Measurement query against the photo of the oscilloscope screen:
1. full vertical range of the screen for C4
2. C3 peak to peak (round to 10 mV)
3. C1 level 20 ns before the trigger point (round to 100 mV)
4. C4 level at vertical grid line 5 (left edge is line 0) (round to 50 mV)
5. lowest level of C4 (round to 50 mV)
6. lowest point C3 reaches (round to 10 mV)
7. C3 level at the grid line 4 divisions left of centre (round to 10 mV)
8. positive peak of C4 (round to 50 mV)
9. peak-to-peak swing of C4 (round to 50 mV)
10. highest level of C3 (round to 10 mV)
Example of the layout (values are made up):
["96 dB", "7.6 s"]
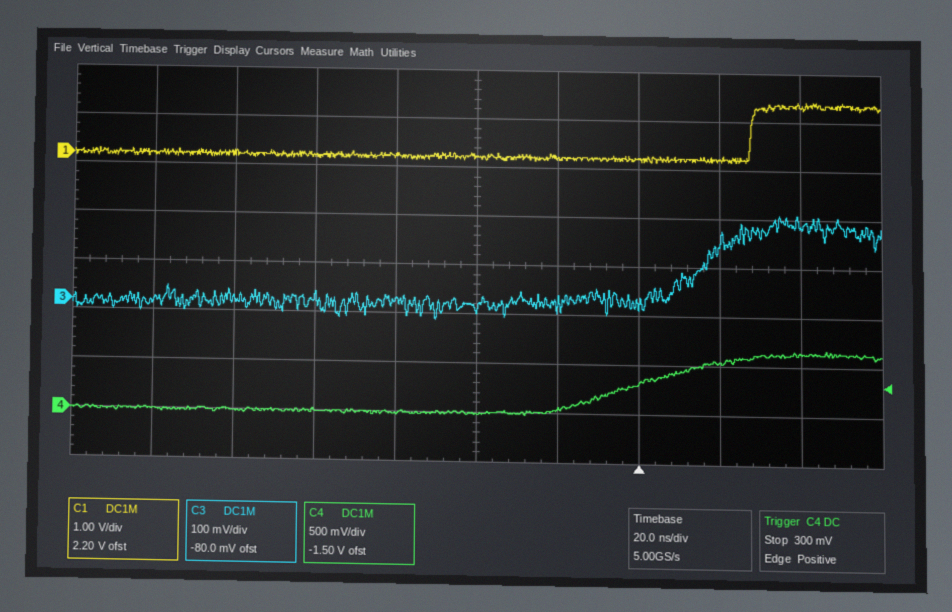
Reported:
["4 V", "220 mV", "0.0 V", "0 mV", "-50 mV", "-30 mV", "0 mV", "650 mV", "700 mV", "190 mV"]
